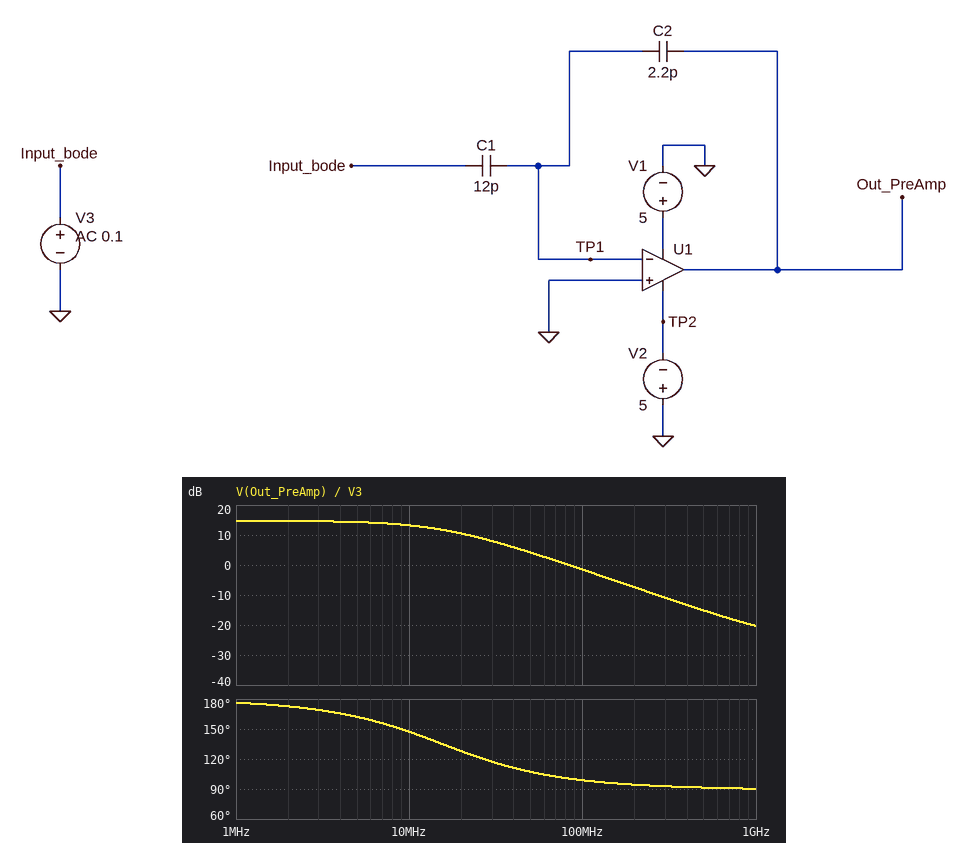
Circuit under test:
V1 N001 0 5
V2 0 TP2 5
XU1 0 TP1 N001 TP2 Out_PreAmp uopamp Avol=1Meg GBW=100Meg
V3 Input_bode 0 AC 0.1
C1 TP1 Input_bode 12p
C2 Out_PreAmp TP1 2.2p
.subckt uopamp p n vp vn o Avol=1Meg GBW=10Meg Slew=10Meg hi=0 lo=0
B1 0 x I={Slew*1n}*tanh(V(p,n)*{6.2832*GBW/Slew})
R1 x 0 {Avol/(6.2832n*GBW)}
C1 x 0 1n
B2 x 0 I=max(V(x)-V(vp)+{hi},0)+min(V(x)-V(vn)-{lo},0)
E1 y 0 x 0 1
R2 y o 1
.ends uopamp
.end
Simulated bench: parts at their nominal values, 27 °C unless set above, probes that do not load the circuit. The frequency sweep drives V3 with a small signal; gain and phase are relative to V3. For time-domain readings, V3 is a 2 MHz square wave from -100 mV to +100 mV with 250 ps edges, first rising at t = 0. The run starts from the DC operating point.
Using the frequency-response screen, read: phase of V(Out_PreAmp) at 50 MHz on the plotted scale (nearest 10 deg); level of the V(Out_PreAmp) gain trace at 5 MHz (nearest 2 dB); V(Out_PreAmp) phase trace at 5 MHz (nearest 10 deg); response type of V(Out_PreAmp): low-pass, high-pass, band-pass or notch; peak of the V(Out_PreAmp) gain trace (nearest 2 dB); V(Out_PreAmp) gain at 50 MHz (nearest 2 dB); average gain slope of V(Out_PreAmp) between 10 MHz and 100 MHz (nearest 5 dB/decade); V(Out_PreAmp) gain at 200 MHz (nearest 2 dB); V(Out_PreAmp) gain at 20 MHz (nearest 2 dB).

110 deg
14 dB
160 deg
low-pass
14 dB
4 dB
-15 dB/decade
-8 dB
10 dB
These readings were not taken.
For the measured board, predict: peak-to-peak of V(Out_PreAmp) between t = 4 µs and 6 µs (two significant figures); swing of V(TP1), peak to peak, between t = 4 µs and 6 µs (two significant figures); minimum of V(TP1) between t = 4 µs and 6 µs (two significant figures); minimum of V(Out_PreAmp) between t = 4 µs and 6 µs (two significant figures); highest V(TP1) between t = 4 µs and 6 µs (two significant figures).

1.1 V
340 mV
-170 mV
-1.1 V
170 mV
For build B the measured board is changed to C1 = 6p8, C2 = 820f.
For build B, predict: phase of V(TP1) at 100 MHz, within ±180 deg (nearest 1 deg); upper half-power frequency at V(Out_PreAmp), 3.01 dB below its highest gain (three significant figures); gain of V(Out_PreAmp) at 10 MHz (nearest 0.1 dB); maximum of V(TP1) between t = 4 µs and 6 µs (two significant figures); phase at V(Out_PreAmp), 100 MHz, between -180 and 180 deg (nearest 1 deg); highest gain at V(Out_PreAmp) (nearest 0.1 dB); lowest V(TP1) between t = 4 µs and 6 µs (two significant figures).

6 deg
10.8 MHz
15.7 dB
180 mV
96 deg
18.4 dB
-180 mV
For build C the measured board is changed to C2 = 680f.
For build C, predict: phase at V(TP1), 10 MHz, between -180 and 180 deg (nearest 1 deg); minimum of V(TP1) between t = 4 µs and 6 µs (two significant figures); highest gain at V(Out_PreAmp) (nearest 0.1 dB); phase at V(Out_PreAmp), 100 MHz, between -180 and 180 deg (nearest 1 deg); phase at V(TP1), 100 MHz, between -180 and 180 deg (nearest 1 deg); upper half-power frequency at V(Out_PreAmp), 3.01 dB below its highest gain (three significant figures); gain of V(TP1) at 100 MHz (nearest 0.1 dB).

28 deg
-160 mV
24.9 dB
93 deg
3 deg
5.36 MHz
-0.5 dB
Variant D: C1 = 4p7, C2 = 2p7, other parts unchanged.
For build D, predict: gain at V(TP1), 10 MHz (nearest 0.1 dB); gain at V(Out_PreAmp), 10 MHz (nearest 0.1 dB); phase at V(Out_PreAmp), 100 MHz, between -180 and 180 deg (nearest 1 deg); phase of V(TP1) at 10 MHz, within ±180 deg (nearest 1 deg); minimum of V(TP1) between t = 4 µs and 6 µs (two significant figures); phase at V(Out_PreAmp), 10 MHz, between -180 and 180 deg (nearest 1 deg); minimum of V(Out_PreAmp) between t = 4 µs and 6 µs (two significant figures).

-15.5 dB
4.5 dB
110 deg
75 deg
-130 mV
165 deg
-350 mV
